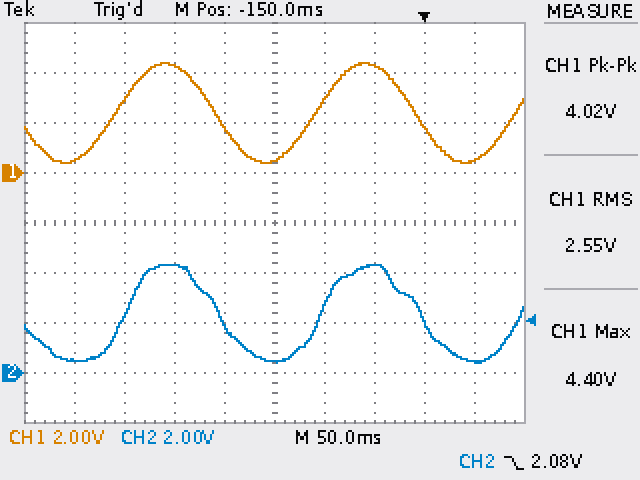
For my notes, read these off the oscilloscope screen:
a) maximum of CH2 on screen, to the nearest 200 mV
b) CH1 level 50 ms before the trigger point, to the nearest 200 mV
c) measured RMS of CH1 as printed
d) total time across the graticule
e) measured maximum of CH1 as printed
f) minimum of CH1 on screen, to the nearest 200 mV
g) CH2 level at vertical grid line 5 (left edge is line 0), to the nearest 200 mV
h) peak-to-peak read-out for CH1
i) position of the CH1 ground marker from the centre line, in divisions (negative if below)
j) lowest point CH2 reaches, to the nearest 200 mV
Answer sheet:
4.4 V
4.2 V
2.55 V
500 ms
4.40 V
400 mV
400 mV
4.02 V
+1.0 div
400 mV
